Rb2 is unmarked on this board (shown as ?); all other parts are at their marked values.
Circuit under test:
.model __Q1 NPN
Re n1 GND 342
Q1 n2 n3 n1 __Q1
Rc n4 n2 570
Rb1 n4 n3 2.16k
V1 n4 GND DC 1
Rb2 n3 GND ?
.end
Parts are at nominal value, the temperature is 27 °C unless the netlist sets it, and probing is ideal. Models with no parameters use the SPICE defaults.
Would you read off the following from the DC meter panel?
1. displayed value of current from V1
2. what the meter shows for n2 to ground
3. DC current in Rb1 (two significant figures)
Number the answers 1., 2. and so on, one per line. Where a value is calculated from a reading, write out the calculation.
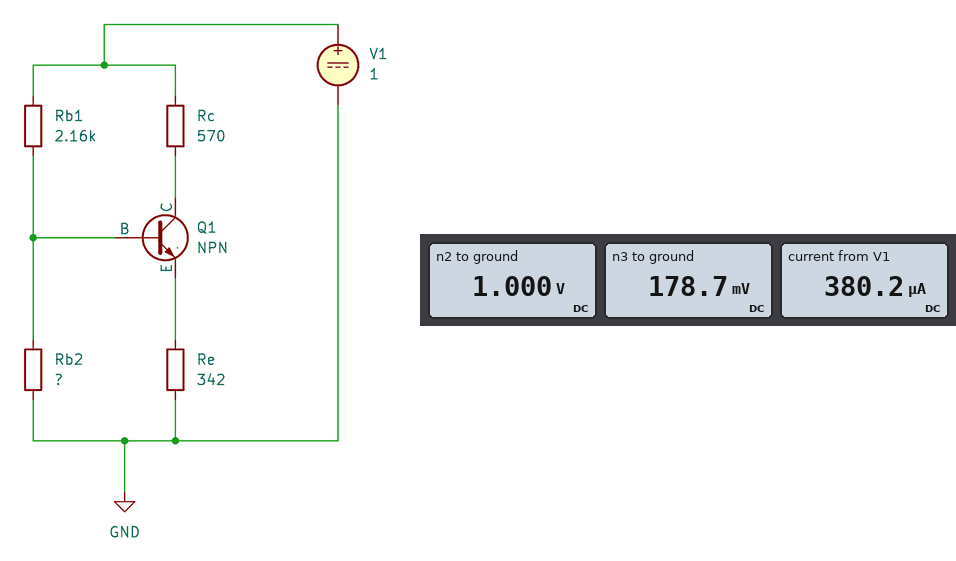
1. 380.2 µA
2. 1.000 V
3. (1 V - 178.7 mV) / 2.16 kΩ = 380 µA
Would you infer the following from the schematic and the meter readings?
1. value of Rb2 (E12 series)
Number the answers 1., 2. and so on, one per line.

1. 470 Ω
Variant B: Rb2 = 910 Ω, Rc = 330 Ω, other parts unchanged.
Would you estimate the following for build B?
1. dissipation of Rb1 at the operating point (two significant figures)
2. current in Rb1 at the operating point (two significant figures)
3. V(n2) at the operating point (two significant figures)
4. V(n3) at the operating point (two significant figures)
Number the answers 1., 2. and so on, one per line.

1. 230 µW
2. 330 µA
3. 1.0 V
4. 300 mV
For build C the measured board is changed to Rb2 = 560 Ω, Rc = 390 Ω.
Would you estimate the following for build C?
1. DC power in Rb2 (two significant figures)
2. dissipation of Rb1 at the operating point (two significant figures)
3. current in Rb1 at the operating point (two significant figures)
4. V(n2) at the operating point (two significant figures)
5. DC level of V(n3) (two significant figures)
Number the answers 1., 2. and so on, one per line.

1. 76 µW
2. 290 µW
3. 370 µA
4. 1.0 V
5. 210 mV
